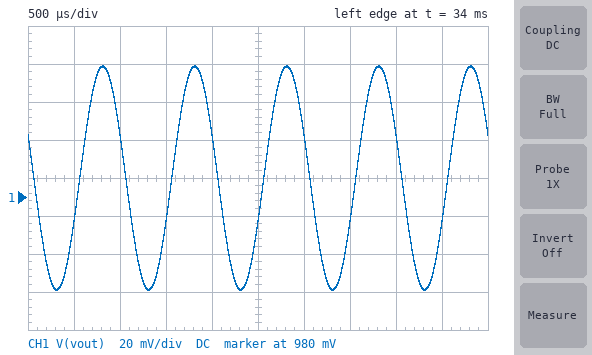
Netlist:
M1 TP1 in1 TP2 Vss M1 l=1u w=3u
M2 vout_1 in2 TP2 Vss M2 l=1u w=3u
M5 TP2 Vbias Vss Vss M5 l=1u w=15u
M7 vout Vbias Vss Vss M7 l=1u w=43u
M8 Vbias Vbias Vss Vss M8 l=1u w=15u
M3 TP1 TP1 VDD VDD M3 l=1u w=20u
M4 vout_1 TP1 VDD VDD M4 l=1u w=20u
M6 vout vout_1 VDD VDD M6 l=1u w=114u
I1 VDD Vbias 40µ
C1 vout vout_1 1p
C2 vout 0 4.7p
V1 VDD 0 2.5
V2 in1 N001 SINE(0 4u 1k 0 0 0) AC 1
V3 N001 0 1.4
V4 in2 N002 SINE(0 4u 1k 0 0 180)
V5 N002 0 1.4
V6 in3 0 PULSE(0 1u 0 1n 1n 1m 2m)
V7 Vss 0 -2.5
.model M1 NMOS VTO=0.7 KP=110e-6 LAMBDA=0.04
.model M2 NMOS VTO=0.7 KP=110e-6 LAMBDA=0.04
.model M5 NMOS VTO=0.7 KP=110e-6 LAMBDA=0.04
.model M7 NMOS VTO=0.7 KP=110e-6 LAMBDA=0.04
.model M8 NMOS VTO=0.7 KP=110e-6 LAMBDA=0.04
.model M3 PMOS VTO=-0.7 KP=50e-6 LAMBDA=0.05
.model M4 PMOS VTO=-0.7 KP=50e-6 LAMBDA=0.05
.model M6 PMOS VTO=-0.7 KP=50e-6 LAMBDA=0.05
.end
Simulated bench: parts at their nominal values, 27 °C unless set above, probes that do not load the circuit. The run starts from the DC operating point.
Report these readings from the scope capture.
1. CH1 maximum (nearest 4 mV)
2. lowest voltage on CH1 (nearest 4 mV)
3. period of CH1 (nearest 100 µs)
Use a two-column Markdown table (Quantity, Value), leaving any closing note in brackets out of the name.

| Quantity | Value |
|---|---|
| CH1 maximum | 1.048 V |
| lowest voltage on CH1 | 932 mV |
| period of CH1 | 1.0 ms |
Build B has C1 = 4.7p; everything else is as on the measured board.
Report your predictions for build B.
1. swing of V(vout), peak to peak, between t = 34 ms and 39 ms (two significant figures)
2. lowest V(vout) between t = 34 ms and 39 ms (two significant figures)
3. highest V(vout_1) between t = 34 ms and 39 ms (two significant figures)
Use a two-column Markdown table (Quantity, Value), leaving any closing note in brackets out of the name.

| Quantity | Value |
|---|---|
| swing of V(vout), peak to peak, between t = 34 ms and 39 ms | 58 mV |
| lowest V(vout) between t = 34 ms and 39 ms | 960 mV |
| highest V(vout_1) between t = 34 ms and 39 ms | 1.6 V |
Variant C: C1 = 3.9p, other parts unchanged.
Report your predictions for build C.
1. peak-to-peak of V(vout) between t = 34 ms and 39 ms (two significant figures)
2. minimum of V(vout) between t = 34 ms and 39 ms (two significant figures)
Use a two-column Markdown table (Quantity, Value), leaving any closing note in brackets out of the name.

| Quantity | Value |
|---|---|
| peak-to-peak of V(vout) between t = 34 ms and 39 ms | 67 mV |
| minimum of V(vout) between t = 34 ms and 39 ms | 960 mV |
